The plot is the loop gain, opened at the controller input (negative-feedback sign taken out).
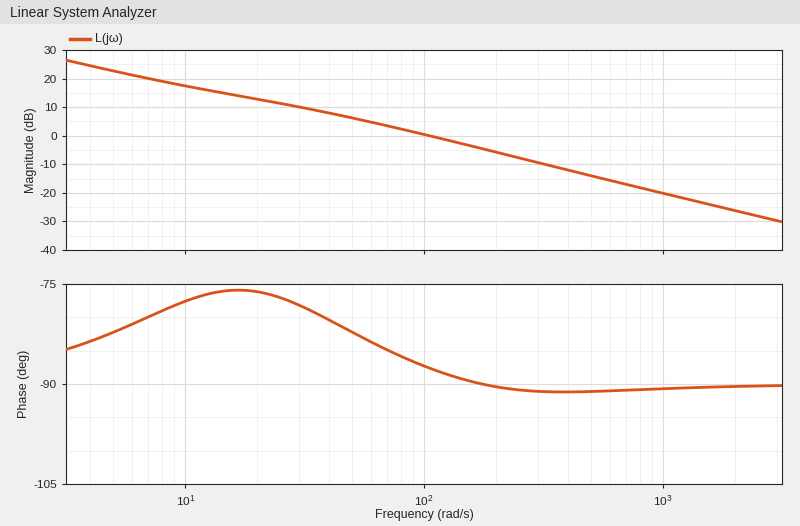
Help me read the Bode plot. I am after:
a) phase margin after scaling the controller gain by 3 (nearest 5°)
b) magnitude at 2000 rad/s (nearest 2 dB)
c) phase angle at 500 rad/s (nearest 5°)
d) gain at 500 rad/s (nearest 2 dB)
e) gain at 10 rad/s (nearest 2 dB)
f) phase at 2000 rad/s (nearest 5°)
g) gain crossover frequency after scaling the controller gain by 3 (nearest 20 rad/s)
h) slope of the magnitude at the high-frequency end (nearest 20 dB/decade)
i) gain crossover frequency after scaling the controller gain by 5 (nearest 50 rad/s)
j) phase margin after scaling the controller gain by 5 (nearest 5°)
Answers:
90°
-26 dB
-90°
-14 dB
18 dB
-90°
300 rad/s
-20 dB/decade
500 rad/s
90°
